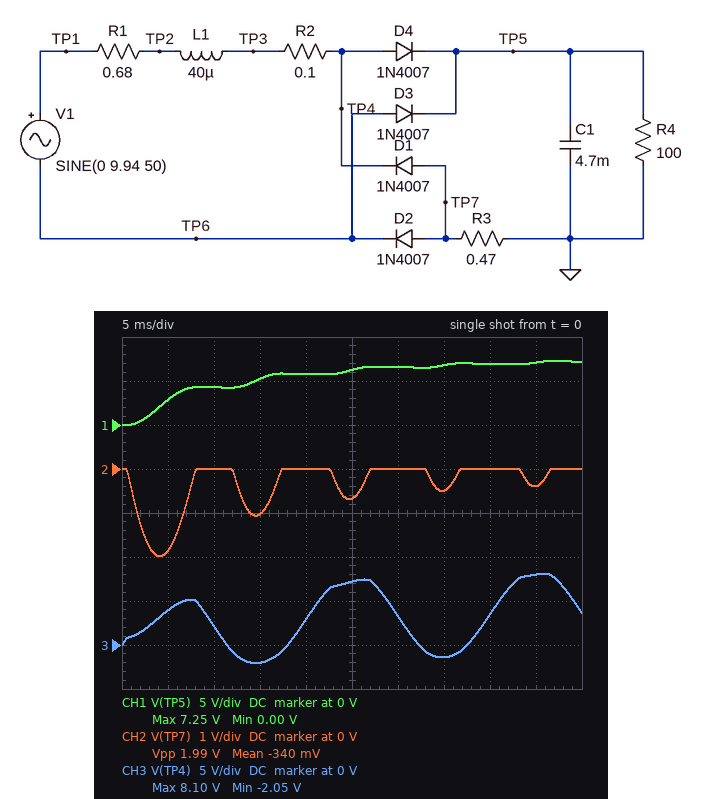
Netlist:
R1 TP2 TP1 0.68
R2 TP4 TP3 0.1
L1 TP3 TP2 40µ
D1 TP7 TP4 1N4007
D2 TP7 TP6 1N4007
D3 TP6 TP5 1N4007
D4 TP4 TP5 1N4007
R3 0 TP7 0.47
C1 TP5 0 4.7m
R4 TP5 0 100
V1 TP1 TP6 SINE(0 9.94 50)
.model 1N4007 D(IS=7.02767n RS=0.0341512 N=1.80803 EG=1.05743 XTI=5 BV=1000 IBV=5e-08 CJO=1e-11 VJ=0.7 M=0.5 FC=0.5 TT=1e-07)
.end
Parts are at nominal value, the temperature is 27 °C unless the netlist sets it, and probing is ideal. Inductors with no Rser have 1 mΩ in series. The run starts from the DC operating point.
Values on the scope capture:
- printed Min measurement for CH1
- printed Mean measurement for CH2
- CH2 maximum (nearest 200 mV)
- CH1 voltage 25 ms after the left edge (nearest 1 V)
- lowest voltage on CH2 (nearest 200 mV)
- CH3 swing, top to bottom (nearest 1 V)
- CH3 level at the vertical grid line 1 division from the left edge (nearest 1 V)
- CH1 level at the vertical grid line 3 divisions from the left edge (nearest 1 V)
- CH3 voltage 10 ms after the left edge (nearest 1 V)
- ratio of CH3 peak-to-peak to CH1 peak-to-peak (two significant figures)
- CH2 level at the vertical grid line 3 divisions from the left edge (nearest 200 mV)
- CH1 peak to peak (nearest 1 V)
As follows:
0.00 V
-340 mV
0 V
6 V
-2.0 V
10 V
4 V
5 V
2 V
1.4
-1.0 V
7 V
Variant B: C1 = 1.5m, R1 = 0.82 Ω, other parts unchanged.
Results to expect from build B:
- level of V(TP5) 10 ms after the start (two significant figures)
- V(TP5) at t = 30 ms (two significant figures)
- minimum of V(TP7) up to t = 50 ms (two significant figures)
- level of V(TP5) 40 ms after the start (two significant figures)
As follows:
6.5 V
7.5 V
-1.2 V
7.6 V
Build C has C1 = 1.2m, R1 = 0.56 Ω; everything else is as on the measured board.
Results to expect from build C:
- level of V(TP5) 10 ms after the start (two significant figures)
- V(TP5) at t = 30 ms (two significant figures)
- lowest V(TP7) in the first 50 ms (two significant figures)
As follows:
7.1 V
7.6 V
-1.1 V
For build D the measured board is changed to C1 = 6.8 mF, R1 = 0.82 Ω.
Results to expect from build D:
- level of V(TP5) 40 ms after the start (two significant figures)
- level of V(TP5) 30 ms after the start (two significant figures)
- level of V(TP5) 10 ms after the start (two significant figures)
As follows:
6.2 V
5.7 V
3.2 V
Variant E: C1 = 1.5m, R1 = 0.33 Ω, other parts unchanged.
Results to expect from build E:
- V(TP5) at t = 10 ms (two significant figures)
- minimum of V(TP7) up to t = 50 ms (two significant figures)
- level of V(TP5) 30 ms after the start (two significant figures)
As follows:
7.2 V
-1.4 V
7.7 V
